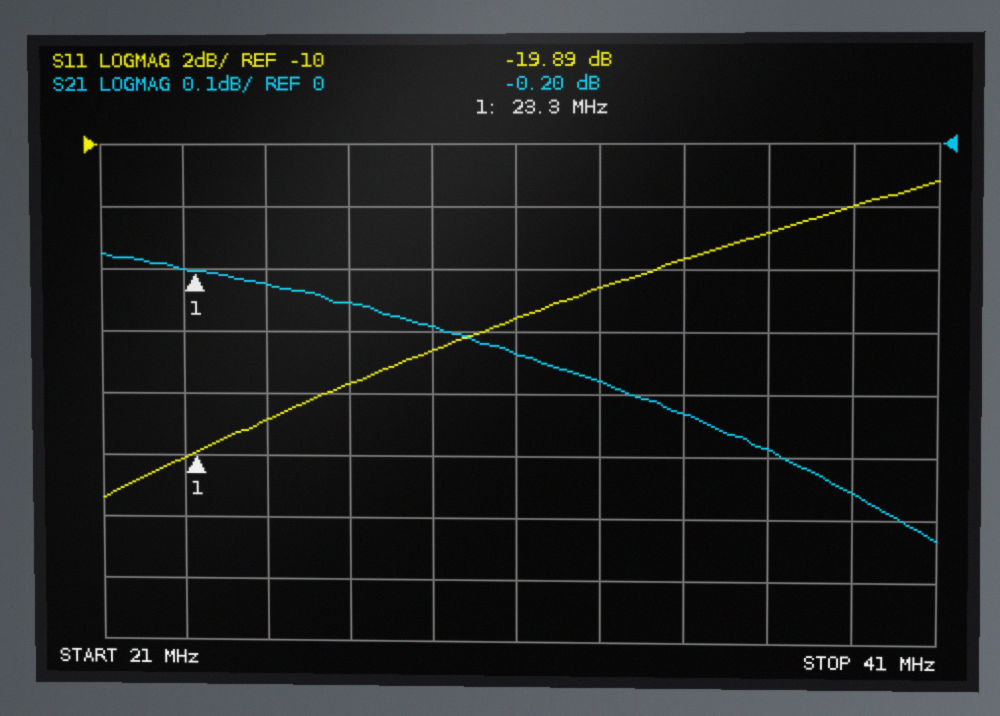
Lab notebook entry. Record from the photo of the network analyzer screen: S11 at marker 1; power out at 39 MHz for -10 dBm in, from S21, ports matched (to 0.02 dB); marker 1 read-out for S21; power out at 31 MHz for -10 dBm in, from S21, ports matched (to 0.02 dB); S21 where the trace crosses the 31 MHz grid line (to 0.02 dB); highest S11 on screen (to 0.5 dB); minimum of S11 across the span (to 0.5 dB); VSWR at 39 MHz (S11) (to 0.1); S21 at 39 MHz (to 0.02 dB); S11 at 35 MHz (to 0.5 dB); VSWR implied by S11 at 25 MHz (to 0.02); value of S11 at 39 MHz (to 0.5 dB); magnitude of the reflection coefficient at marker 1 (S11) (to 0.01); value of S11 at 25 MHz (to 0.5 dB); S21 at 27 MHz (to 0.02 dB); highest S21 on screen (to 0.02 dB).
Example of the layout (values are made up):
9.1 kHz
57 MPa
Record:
-19.89 dB
-10.56 dBm
-0.20 dB
-10.34 dBm
-0.34 dB
-11.0 dB
-21.5 dB
1.7
-0.56 dB
-13.5 dB
1.26
-12.0 dB
0.10
-19.0 dB
-0.26 dB
-0.18 dB
